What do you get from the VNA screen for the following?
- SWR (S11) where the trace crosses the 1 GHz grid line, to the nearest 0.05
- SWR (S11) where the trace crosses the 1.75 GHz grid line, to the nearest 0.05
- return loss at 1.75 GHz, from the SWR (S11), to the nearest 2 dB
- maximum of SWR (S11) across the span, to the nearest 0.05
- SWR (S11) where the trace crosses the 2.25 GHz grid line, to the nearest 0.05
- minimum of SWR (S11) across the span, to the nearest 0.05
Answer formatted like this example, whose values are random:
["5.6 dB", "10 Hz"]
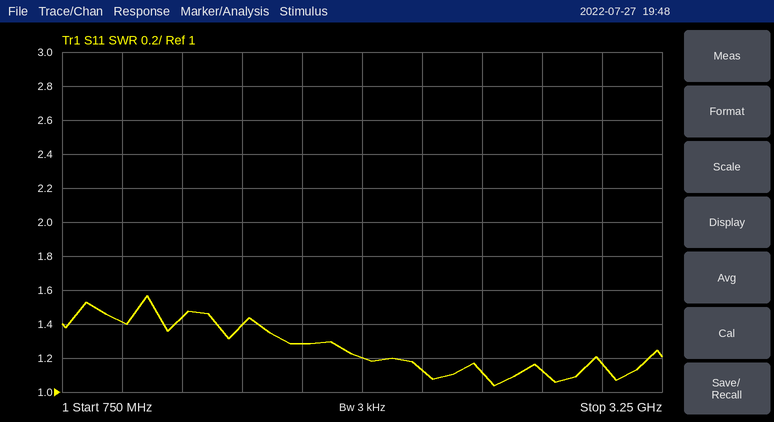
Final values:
["1.40", "1.30", "18 dB", "1.55", "1.15", "1.05"]
